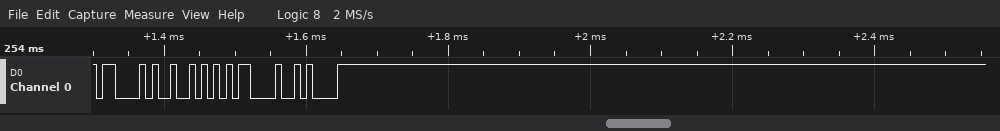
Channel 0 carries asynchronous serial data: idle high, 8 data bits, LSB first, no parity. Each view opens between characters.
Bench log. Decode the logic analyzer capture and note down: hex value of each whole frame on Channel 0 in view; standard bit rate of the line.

43, 52, 0D, 0A
115200 baud
